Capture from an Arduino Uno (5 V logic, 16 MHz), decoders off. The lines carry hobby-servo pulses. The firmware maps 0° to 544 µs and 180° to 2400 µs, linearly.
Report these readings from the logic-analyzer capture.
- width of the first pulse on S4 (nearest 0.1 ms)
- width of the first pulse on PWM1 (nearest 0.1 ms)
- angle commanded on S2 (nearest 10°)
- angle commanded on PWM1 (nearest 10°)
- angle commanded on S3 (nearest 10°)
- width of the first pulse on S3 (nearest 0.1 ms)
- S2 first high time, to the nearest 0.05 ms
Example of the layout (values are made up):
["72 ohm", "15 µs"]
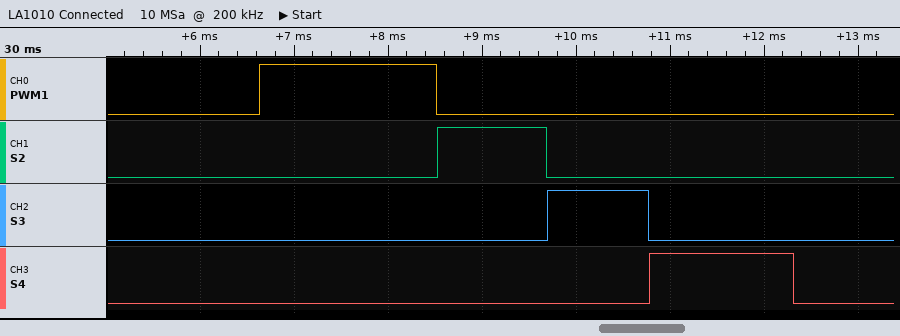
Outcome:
["1.5 ms", "1.9 ms", "60°", "130°", "50°", "1.1 ms", "1.15 ms"]
